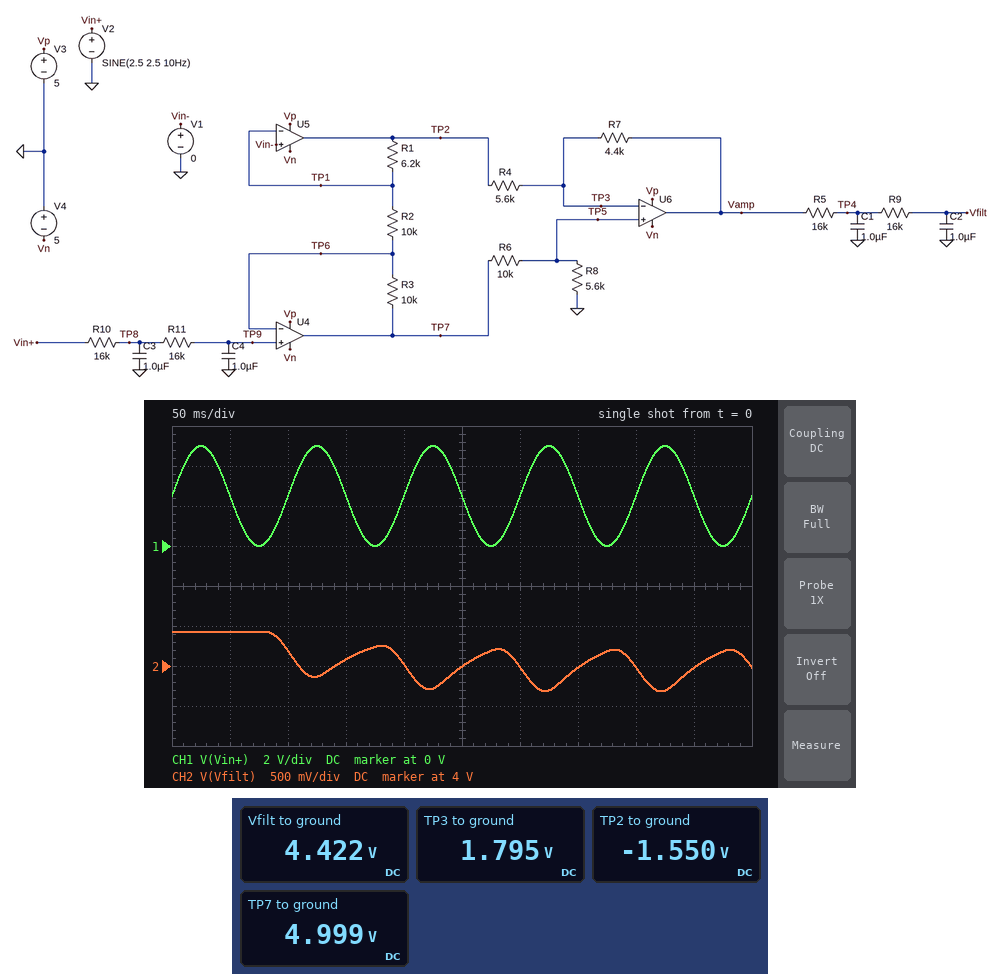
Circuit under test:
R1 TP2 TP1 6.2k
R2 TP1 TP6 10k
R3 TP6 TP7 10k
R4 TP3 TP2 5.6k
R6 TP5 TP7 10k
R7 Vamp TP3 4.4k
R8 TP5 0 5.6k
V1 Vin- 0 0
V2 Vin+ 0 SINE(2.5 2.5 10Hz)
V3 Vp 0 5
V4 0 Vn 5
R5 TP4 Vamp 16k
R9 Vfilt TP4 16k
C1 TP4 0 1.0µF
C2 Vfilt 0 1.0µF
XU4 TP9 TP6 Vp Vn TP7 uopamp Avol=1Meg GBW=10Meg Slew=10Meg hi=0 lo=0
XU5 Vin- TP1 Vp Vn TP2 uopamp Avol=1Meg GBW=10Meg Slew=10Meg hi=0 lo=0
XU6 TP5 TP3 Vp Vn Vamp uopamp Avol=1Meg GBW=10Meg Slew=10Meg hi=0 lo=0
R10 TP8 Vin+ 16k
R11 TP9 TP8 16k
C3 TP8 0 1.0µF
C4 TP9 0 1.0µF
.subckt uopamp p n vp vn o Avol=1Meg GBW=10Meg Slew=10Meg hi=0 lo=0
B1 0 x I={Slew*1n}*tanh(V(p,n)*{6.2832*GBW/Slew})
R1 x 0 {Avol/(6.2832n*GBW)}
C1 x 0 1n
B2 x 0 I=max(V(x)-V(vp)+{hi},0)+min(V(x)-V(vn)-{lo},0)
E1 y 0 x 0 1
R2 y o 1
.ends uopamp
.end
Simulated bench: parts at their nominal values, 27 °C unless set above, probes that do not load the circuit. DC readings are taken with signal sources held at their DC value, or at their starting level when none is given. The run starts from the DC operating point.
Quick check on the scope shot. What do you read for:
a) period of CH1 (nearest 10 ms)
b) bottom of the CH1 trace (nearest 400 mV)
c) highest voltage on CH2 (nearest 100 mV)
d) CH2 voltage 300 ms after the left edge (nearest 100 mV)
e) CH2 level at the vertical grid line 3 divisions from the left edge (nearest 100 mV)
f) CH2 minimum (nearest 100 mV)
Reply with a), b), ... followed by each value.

a) 100 ms
b) 0 V
c) 4.4 V
d) 4.0 V
e) 4.1 V
f) 3.7 V
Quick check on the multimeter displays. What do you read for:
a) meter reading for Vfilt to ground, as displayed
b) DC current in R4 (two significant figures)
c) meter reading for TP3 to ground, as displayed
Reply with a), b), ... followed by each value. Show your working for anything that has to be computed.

a) 4.422 V
b) (1.795 V - (-1.55 V)) / 5.6 kΩ = 600 µA
c) 1.795 V
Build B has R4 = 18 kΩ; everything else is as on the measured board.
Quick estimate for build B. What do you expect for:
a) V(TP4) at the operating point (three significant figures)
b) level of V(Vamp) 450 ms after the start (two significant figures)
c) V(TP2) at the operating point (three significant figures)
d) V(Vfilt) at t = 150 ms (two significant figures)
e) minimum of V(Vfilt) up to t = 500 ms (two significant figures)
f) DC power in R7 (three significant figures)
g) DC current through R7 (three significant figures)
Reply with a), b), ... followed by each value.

a) 2.61 V
b) 2.6 V
c) -1.55 V
d) 2.4 V
e) 2.2 V
f) 152 µW
g) 186 µA
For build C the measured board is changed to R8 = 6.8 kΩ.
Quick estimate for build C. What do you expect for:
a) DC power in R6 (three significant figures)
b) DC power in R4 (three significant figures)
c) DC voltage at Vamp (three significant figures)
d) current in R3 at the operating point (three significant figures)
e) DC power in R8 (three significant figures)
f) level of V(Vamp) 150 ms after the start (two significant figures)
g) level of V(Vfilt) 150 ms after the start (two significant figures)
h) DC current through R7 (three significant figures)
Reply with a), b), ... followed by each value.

a) 886 µW
b) 2.28 mW
c) 4.83 V
d) 250 µA
e) 602 µW
f) 4.8 V
g) 4.5 V
h) 638 µA
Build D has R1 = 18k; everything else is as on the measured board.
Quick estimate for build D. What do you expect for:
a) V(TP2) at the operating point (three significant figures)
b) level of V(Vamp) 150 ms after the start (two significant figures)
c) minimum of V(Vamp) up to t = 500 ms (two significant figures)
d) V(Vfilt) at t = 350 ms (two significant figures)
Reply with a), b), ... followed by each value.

a) -4.50 V
b) 5.0 V
c) 4.5 V
d) 4.9 V
